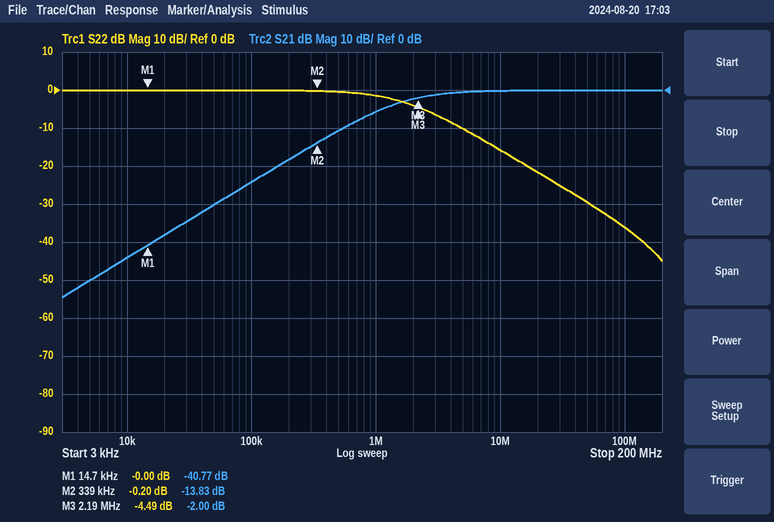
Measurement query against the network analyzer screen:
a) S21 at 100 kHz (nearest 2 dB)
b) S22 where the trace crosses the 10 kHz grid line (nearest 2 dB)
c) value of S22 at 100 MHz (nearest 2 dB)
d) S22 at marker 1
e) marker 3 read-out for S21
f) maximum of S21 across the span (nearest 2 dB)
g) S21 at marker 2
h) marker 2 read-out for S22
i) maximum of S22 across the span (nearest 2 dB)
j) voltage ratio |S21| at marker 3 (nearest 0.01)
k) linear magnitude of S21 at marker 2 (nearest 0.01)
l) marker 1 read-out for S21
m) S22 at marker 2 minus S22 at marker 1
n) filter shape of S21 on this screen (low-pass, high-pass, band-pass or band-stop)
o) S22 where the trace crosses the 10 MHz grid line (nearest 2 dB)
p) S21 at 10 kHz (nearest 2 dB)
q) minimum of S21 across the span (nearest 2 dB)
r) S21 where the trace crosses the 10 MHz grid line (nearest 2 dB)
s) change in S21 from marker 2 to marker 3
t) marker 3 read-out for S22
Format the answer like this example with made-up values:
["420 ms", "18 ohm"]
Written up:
["-24 dB", "0 dB", "-36 dB", "-0.00 dB", "-2.00 dB", "0 dB", "-13.83 dB", "-0.20 dB", "0 dB", "0.79", "0.20", "-40.77 dB", "-0.20 dB", "high-pass", "-16 dB", "-44 dB", "-54 dB", "0 dB", "11.83 dB", "-4.49 dB"]
